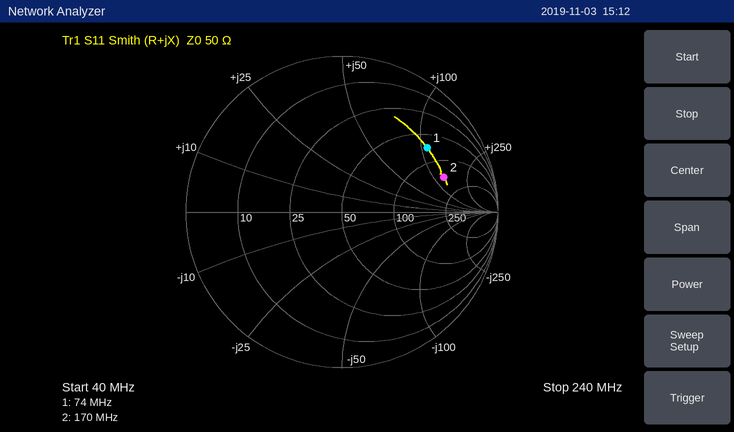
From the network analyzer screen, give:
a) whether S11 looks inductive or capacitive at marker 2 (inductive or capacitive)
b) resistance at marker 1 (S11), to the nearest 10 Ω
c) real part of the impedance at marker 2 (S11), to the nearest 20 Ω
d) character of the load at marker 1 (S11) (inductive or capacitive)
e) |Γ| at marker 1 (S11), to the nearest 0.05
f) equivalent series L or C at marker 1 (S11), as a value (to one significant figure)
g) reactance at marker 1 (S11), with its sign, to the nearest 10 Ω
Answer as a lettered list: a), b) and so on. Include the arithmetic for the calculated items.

a) inductive
b) 70 Ω
c) 160 Ω
d) inductive
e) 0.70
f) L = 110 Ω/(2π × 74 MHz) ≈ 237 nH, so 200 nH to one significant figure
g) +110 Ω
